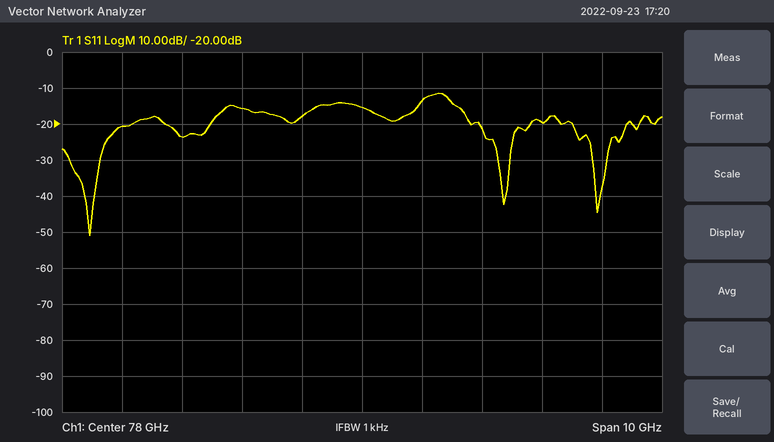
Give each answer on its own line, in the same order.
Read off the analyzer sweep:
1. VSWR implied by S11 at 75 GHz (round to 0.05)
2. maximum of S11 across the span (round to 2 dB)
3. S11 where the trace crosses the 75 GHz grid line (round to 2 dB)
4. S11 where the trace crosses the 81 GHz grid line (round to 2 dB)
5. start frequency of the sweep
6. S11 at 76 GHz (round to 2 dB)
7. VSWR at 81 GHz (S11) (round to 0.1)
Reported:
1.15
-12 dB
-24 dB
-20 dB
73 GHz
-16 dB
1.2
